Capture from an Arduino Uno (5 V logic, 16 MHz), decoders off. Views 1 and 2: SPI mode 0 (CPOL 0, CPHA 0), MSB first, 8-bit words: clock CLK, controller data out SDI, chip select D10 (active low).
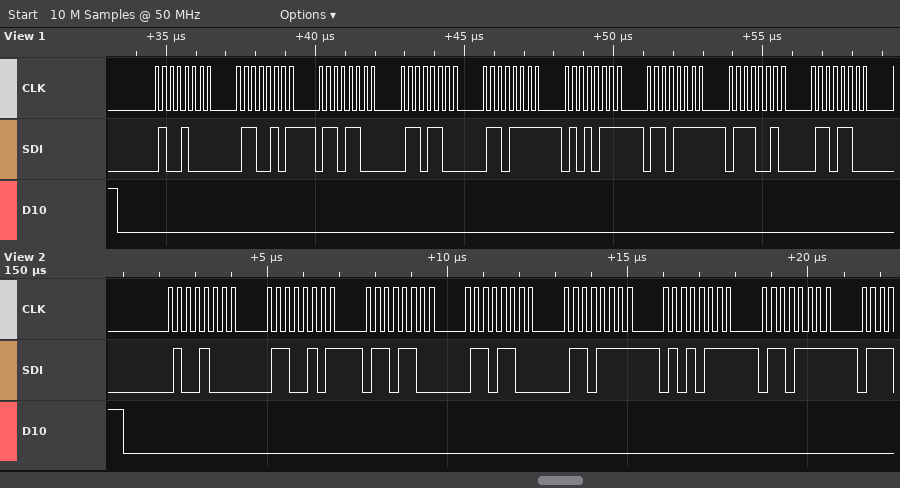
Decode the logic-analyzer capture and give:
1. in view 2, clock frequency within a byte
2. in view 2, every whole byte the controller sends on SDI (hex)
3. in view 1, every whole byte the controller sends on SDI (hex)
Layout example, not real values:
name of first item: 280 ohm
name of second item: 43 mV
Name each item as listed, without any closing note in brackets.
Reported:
in view 2, clock frequency within a byte: 4 MHz
in view 2, every whole byte the controller sends on SDI: 0x48 0x65 0x6C 0x6C 0x6F 0x57 0x6F
in view 1, every whole byte the controller sends on SDI: 48 65 6C 6C 6F 57 6F 72 6C
